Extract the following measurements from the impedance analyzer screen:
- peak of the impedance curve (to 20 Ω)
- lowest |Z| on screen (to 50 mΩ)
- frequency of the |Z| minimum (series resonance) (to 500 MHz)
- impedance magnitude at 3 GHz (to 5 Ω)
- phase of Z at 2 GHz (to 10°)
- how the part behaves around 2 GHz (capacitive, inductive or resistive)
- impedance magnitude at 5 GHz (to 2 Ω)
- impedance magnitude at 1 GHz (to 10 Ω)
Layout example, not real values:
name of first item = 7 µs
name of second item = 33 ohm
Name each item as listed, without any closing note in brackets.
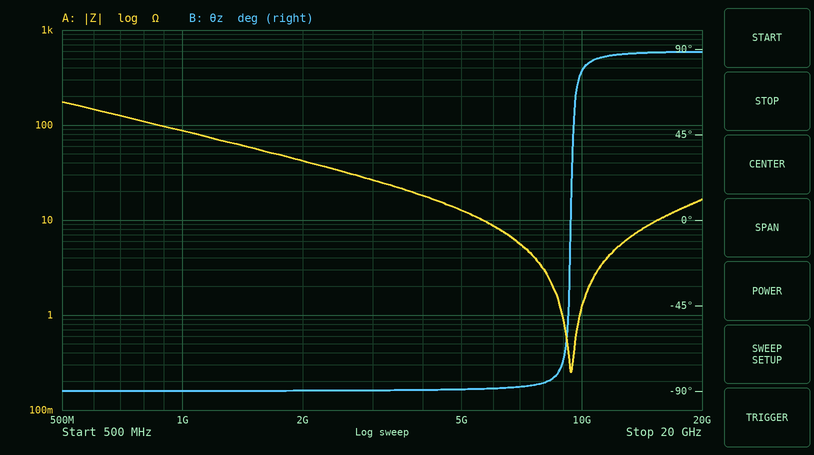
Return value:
peak of the impedance curve = 180 Ω
lowest |Z| on screen = 250 mΩ
frequency of the |Z| minimum (series resonance) = 9.5 GHz
impedance magnitude at 3 GHz = 25 Ω
phase of Z at 2 GHz = -90°
how the part behaves around 2 GHz = capacitive
impedance magnitude at 5 GHz = 12 Ω
impedance magnitude at 1 GHz = 90 Ω
